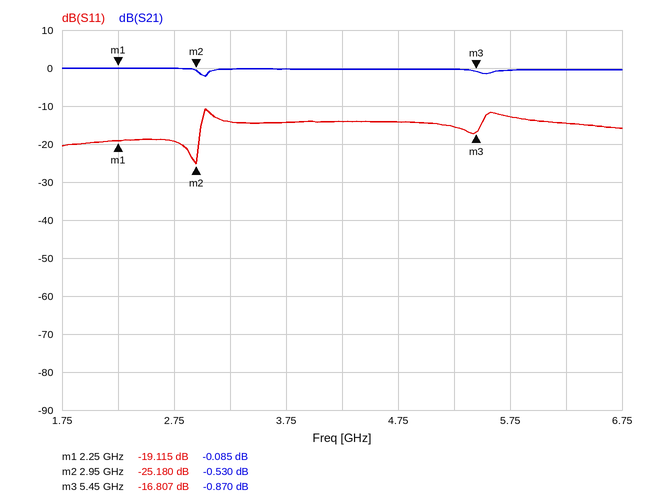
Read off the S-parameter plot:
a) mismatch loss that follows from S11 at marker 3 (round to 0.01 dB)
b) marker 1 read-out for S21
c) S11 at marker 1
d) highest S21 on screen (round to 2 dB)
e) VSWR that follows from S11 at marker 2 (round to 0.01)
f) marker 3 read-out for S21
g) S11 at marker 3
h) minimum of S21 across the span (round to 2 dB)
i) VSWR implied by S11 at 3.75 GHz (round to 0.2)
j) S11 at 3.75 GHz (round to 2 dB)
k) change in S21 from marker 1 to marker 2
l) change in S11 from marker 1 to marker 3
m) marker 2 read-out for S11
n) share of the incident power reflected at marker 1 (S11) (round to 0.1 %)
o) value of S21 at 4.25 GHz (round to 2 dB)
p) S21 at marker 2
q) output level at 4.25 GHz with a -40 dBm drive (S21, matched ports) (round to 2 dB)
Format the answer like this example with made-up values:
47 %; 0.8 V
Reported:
0.09 dB; -0.085 dB; -19.115 dB; 0 dB; 1.12; -0.870 dB; -16.807 dB; -2 dB; 1.4; -14 dB; -0.445 dB; 2.308 dB; -25.180 dB; 1.2 %; 0 dB; -0.530 dB; -40 dBm
